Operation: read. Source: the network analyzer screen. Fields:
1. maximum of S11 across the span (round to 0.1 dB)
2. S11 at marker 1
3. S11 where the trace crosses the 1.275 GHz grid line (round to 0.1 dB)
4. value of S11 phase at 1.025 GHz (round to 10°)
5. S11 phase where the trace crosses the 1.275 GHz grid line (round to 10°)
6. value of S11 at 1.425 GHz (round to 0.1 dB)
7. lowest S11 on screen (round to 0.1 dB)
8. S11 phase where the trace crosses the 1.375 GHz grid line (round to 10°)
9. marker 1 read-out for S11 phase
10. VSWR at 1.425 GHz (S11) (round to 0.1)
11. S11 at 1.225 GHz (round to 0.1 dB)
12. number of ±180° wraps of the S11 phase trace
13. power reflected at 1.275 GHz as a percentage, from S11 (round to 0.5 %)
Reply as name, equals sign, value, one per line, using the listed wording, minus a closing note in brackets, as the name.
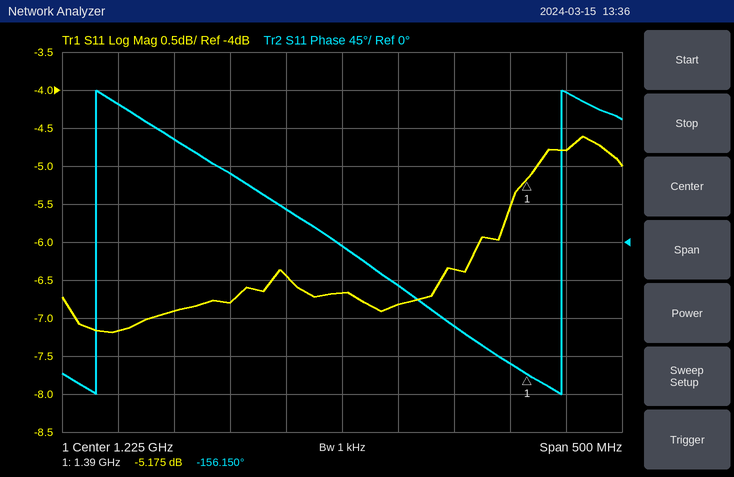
maximum of S11 across the span = -4.6 dB
S11 at marker 1 = -5.175 dB
S11 where the trace crosses the 1.275 GHz grid line = -6.8 dB
value of S11 phase at 1.025 GHz = 160°
S11 phase where the trace crosses the 1.275 GHz grid line = -50°
value of S11 at 1.425 GHz = -4.8 dB
lowest S11 on screen = -7.2 dB
S11 phase where the trace crosses the 1.375 GHz grid line = -140°
marker 1 read-out for S11 phase = -156.150°
VSWR at 1.425 GHz (S11) = 3.7
S11 at 1.225 GHz = -6.7 dB
number of ±180° wraps of the S11 phase trace = 2
power reflected at 1.275 GHz as a percentage, from S11 = 21.0 %
